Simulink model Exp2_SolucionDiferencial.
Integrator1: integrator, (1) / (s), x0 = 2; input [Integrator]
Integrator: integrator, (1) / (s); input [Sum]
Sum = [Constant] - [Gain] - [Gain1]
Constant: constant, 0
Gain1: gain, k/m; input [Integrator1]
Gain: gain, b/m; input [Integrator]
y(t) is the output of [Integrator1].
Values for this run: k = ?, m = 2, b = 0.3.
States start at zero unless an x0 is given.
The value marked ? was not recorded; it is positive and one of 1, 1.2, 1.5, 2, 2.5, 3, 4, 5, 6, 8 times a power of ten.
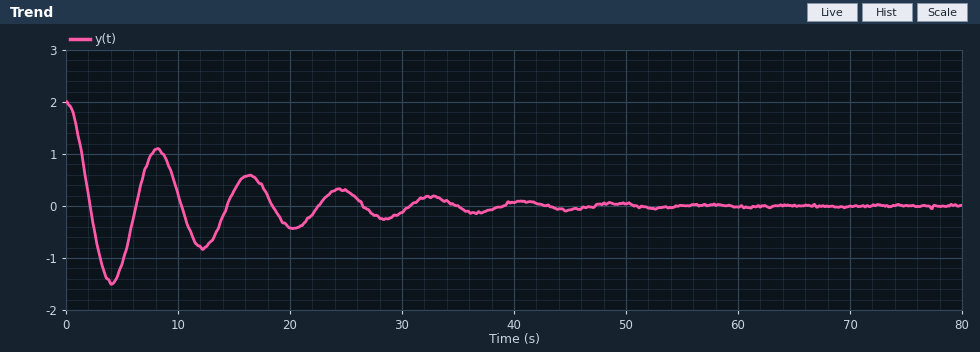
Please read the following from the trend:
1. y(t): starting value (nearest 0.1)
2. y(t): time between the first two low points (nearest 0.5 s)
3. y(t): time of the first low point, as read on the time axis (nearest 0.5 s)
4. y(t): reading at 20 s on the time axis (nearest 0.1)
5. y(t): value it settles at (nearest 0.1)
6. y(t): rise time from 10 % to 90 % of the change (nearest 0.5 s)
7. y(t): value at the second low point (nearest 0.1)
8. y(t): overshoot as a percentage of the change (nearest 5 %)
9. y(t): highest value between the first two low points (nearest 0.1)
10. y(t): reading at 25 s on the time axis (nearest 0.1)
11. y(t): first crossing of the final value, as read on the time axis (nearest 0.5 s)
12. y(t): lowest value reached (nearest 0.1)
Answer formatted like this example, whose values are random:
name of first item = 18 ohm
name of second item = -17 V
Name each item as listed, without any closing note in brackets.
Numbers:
y(t): starting value = 2.0
y(t): time between the first two low points = 8.0 s
y(t): time of the first low point, as read on the time axis = 4.0 s
y(t): reading at 20 s on the time axis = -0.4
y(t): value it settles at = 0.0
y(t): rise time from 10 % to 90 % of the change = 1.5 s
y(t): value at the second low point = -0.8
y(t): overshoot as a percentage of the change = 75 %
y(t): highest value between the first two low points = 1.1
y(t): reading at 25 s on the time axis = 0.3
y(t): first crossing of the final value, as read on the time axis = 2.0 s
y(t): lowest value reached = -1.5
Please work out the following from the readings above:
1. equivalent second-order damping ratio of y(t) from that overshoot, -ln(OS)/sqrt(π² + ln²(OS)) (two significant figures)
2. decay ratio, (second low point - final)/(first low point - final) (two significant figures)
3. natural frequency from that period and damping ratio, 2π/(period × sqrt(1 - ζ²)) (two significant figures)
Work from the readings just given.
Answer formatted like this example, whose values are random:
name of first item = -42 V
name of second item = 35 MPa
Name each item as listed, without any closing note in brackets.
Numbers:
equivalent second-order damping ratio of y(t) from that overshoot, -ln(OS)/sqrt(π² + ln²(OS)) = 0.091
decay ratio, (second low point - final)/(first low point - final) = 0.53
natural frequency from that period and damping ratio, 2π/(period × sqrt(1 - ζ²)) = 0.79 rad/s
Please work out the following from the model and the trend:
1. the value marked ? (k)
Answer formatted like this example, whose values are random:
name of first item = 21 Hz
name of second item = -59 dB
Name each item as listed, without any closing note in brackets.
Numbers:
the value marked ? = 1.2
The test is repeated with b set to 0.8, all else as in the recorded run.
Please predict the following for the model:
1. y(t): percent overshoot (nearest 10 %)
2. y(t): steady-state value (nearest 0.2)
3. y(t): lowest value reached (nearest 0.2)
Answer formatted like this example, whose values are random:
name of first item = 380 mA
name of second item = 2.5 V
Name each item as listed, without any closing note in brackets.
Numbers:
y(t): percent overshoot = 40 %
y(t): steady-state value = 0.0
y(t): lowest value reached = -0.8
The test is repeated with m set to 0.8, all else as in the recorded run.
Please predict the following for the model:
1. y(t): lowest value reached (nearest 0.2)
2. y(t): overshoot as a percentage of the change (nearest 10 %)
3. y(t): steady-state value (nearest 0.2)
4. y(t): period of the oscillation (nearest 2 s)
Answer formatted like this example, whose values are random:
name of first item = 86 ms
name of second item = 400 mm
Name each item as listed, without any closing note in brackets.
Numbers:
y(t): lowest value reached = -1.2
y(t): overshoot as a percentage of the change = 60 %
y(t): steady-state value = 0.0
y(t): period of the oscillation = 6 s
